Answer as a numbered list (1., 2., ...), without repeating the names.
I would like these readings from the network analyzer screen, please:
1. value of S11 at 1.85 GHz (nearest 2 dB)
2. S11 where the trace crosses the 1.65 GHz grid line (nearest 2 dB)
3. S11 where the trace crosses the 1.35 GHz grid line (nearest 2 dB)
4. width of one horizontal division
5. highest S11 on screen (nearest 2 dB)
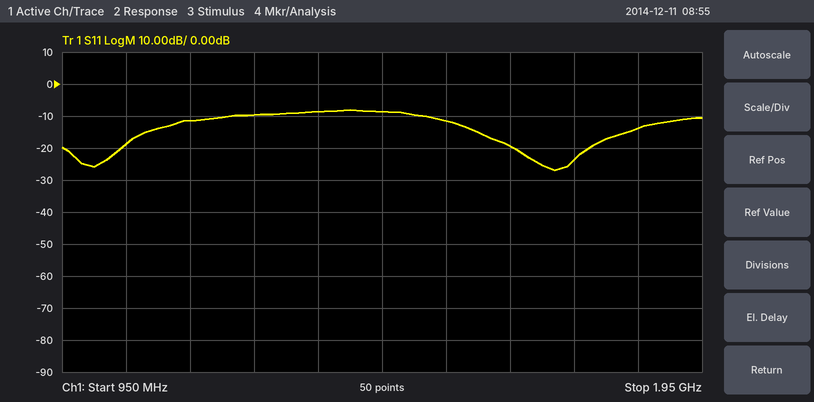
1. -14 dB
2. -20 dB
3. -8 dB
4. 100 MHz
5. -8 dB
